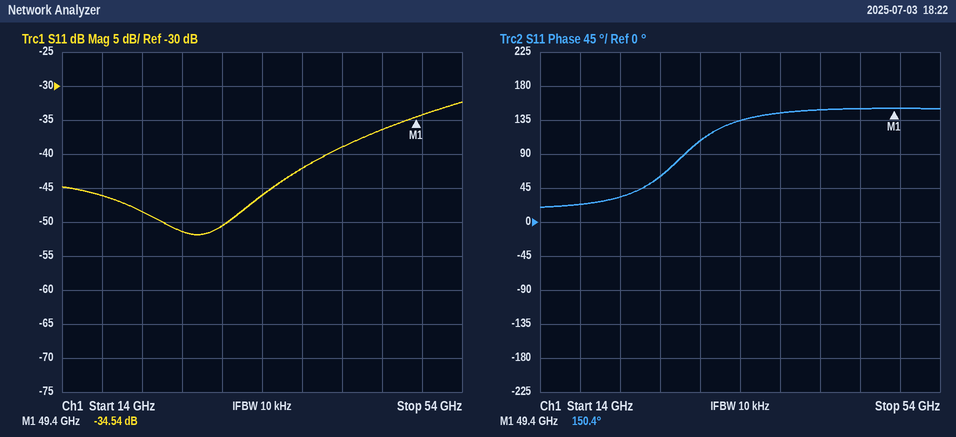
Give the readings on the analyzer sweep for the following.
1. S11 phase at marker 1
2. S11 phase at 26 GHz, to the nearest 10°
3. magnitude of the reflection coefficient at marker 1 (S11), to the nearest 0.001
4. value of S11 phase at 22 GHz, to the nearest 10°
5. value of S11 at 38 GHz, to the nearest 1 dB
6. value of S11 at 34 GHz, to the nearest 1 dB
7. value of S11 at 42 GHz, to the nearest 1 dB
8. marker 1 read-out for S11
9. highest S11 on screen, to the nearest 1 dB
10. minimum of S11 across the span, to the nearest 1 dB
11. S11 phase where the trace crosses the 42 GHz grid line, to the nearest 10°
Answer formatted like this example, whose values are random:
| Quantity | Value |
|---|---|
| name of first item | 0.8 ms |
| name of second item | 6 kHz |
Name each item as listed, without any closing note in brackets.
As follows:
| Quantity | Value |
|---|---|
| S11 phase at marker 1 | 150.4° |
| S11 phase at 26 GHz, to the nearest 10° | 60° |
| magnitude of the reflection coefficient at marker 1 (S11), to the nearest 0.001 | 0.019 |
| value of S11 phase at 22 GHz, to the nearest 10° | 30° |
| value of S11 at 38 GHz, to the nearest 1 dB | -42 dB |
| value of S11 at 34 GHz, to the nearest 1 dB | -46 dB |
| value of S11 at 42 GHz, to the nearest 1 dB | -39 dB |
| marker 1 read-out for S11 | -34.54 dB |
| highest S11 on screen, to the nearest 1 dB | -32 dB |
| minimum of S11 across the span, to the nearest 1 dB | -52 dB |
| S11 phase where the trace crosses the 42 GHz grid line, to the nearest 10° | 150° |
